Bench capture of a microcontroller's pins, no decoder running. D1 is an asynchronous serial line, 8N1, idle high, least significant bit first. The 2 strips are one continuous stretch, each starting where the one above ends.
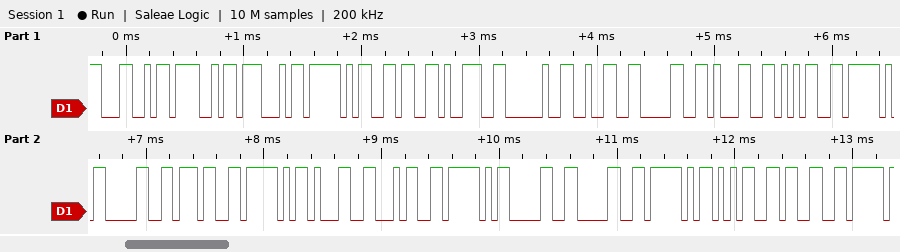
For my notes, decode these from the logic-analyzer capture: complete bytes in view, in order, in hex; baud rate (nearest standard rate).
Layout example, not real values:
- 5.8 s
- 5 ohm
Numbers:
- 0x4C 0x4F 0x47 0x5F 0x36 0x39 0x20 0x32 0x30 0x31 0x35 0x5F 0x30 0x37 0x5F 0x31 0x34 0x5F 0x30 0x30 0x5F 0x35 0x33
- 19200 baud
